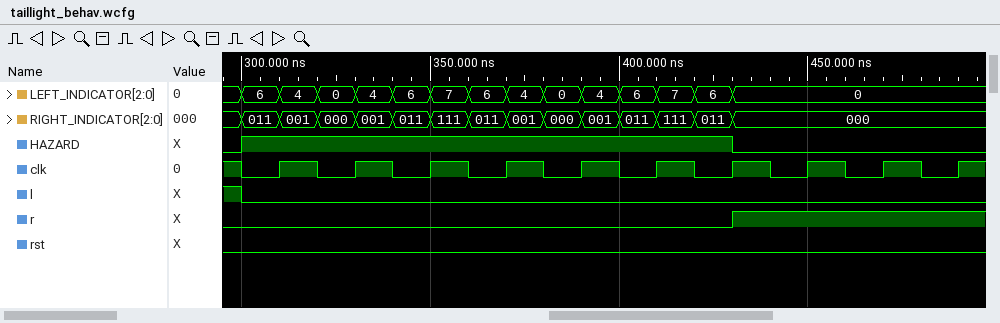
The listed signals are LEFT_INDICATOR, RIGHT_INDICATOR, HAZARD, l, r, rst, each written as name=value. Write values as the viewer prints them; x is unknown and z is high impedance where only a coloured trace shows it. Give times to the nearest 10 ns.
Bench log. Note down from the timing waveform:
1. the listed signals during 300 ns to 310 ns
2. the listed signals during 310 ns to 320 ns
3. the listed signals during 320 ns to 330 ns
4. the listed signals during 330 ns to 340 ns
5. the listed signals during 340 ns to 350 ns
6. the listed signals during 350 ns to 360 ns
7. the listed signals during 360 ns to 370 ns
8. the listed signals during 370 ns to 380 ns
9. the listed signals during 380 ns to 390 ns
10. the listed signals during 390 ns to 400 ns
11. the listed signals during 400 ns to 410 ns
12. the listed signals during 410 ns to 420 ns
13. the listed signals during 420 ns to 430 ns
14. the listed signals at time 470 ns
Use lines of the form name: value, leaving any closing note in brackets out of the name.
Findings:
the listed signals during 300 ns to 310 ns: LEFT_INDICATOR=6, RIGHT_INDICATOR=011, HAZARD=1, l=0, r=0, rst=0
the listed signals during 310 ns to 320 ns: LEFT_INDICATOR=4, RIGHT_INDICATOR=001, HAZARD=1, l=0, r=0, rst=0
the listed signals during 320 ns to 330 ns: LEFT_INDICATOR=0, RIGHT_INDICATOR=000, HAZARD=1, l=0, r=0, rst=0
the listed signals during 330 ns to 340 ns: LEFT_INDICATOR=4, RIGHT_INDICATOR=001, HAZARD=1, l=0, r=0, rst=0
the listed signals during 340 ns to 350 ns: LEFT_INDICATOR=6, RIGHT_INDICATOR=011, HAZARD=1, l=0, r=0, rst=0
the listed signals during 350 ns to 360 ns: LEFT_INDICATOR=7, RIGHT_INDICATOR=111, HAZARD=1, l=0, r=0, rst=0
the listed signals during 360 ns to 370 ns: LEFT_INDICATOR=6, RIGHT_INDICATOR=011, HAZARD=1, l=0, r=0, rst=0
the listed signals during 370 ns to 380 ns: LEFT_INDICATOR=4, RIGHT_INDICATOR=001, HAZARD=1, l=0, r=0, rst=0
the listed signals during 380 ns to 390 ns: LEFT_INDICATOR=0, RIGHT_INDICATOR=000, HAZARD=1, l=0, r=0, rst=0
the listed signals during 390 ns to 400 ns: LEFT_INDICATOR=4, RIGHT_INDICATOR=001, HAZARD=1, l=0, r=0, rst=0
the listed signals during 400 ns to 410 ns: LEFT_INDICATOR=6, RIGHT_INDICATOR=011, HAZARD=1, l=0, r=0, rst=0
the listed signals during 410 ns to 420 ns: LEFT_INDICATOR=7, RIGHT_INDICATOR=111, HAZARD=1, l=0, r=0, rst=0
the listed signals during 420 ns to 430 ns: LEFT_INDICATOR=6, RIGHT_INDICATOR=011, HAZARD=1, l=0, r=0, rst=0
the listed signals at time 470 ns: LEFT_INDICATOR=0, RIGHT_INDICATOR=000, HAZARD=0, l=0, r=1, rst=0
